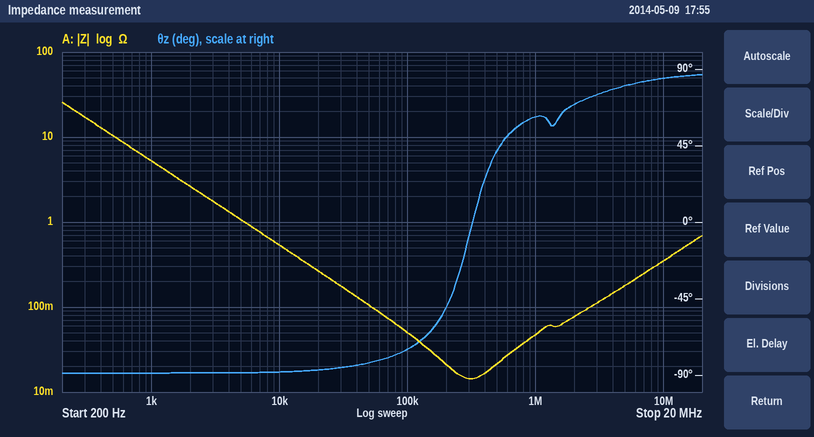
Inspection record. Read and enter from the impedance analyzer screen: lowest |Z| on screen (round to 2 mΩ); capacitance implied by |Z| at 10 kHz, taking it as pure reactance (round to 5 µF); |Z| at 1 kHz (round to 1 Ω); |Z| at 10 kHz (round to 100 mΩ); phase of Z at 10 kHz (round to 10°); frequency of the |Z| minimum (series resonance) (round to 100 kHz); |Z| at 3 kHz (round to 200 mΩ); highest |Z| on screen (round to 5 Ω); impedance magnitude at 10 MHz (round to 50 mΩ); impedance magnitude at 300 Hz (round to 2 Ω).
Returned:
14 mΩ
30 µF
5 Ω
500 mΩ
-90°
300 kHz
1.8 Ω
25 Ω
350 mΩ
18 Ω
